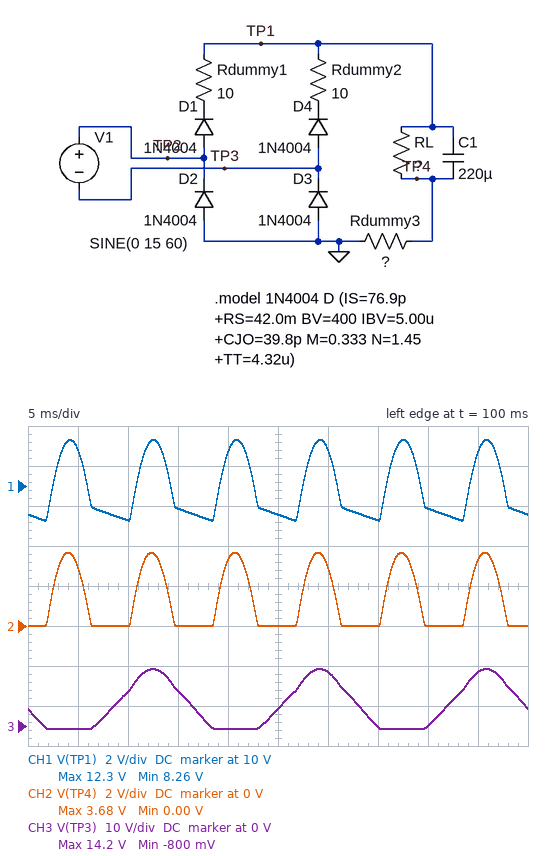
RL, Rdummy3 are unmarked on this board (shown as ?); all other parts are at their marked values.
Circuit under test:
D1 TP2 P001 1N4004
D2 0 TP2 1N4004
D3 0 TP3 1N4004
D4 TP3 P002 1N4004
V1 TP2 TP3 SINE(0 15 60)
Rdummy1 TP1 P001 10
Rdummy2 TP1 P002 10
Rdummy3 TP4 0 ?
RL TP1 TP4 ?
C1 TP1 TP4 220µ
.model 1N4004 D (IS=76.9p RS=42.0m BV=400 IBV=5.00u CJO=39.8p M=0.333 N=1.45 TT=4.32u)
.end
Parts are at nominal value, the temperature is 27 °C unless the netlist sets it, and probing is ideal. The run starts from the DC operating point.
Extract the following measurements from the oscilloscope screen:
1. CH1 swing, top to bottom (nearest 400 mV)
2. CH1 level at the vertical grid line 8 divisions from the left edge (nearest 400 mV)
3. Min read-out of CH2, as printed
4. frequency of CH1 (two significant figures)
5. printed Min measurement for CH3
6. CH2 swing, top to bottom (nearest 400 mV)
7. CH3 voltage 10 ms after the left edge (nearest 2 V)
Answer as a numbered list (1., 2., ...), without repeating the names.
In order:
1. 4.0 V
2. 8.8 V
3. 0.00 V
4. 120 Hz
5. -800 mV
6. 3.6 V
7. 8 V
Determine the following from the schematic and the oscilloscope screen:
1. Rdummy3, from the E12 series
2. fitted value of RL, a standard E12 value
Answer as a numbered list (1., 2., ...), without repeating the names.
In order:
1. 33 Ω
2. 220 Ω
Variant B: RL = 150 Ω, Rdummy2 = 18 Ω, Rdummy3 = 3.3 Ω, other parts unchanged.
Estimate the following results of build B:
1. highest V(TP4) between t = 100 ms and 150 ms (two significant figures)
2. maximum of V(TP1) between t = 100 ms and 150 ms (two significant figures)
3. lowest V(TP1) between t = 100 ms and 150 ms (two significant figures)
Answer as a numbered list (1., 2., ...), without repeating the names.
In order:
1. 850 mV
2. 11 V
3. 8.9 V
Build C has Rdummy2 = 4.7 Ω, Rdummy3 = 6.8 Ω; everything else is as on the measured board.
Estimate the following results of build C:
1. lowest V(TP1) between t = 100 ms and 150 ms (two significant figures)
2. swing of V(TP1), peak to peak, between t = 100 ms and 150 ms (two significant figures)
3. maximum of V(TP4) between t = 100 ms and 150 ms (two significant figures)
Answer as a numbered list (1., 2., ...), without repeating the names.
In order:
1. 10 V
2. 2.4 V
3. 1.5 V
